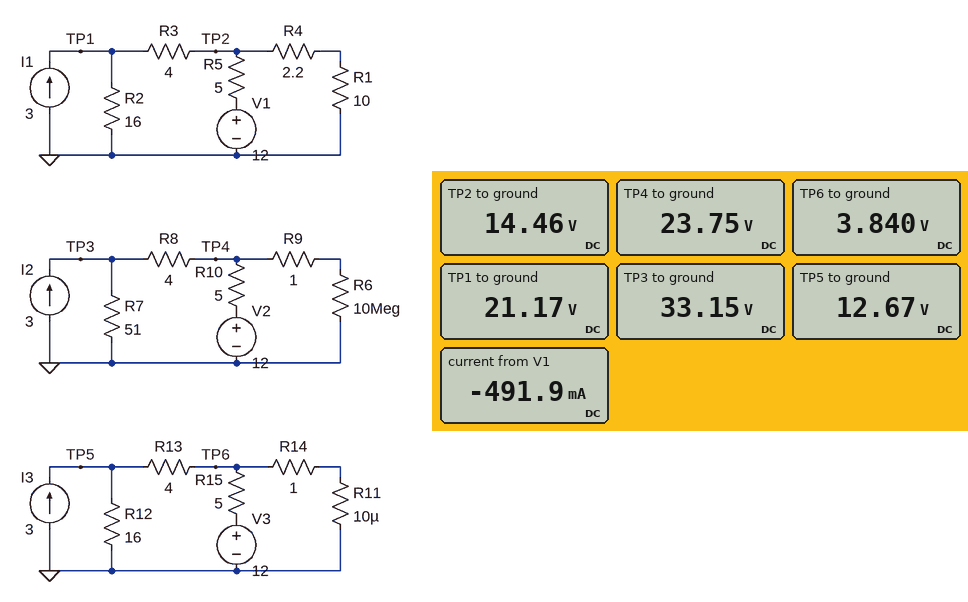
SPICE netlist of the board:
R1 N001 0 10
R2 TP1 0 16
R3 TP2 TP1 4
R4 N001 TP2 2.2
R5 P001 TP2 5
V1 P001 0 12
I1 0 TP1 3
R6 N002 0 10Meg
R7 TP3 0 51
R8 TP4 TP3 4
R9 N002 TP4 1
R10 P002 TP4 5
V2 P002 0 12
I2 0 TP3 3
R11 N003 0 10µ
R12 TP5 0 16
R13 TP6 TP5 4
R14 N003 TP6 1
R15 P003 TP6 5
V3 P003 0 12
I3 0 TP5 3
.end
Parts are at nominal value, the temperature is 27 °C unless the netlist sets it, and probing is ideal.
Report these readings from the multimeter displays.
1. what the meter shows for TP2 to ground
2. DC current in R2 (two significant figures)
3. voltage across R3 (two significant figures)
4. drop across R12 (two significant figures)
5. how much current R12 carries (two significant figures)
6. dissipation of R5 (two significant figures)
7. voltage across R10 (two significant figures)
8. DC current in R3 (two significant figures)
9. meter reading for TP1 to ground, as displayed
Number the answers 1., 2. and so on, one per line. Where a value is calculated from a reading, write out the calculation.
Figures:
1. 14.46 V
2. (21.17 V) / 16 Ω = 1.3 A
3. 21.17 V - 14.46 V = 6.7 V
4. 12.67 V = 13 V
5. (12.67 V) / 16 Ω = 790 mA
6. (14.46 V - 12 V)^2 / 5 Ω = 1.2 W
7. 23.75 V - 12 V = 12 V
8. (21.17 V - 14.46 V) / 4 Ω = 1.7 A
9. 21.17 V
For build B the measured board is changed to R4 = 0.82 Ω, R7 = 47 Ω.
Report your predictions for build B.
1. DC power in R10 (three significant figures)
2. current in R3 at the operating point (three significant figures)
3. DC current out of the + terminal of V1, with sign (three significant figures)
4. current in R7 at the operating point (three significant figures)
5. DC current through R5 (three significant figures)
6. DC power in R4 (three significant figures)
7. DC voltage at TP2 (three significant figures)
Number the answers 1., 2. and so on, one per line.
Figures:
1. 26.5 W
2. 1.70 A
3. -404 mA
4. 696 mA
5. 404 mA
6. 1.38 W
7. 14.0 V
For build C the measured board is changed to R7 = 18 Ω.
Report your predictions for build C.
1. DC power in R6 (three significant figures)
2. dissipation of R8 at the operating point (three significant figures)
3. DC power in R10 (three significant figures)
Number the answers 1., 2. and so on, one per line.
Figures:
1. 39.1 µW
2. 9.68 W
3. 12.1 W
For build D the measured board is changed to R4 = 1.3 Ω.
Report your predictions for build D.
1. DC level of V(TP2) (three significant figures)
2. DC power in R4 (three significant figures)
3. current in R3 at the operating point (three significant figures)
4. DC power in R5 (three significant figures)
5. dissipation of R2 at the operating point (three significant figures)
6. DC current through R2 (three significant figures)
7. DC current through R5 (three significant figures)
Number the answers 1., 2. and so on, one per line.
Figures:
1. 14.2 V
2. 2.05 W
3. 1.69 A
4. 951 mW
5. 27.4 W
6. 1.31 A
7. 436 mA
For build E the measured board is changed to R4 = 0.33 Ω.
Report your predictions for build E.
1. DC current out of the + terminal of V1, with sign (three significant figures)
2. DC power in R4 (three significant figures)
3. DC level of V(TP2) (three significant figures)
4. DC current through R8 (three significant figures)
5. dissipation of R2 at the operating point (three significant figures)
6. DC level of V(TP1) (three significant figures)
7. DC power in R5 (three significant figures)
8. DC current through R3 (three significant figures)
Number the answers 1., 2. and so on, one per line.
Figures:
1. -368 mA
2. 592 mW
3. 13.8 V
4. 2.35 A
5. 26.7 W
6. 20.7 V
7. 678 mW
8. 1.71 A
